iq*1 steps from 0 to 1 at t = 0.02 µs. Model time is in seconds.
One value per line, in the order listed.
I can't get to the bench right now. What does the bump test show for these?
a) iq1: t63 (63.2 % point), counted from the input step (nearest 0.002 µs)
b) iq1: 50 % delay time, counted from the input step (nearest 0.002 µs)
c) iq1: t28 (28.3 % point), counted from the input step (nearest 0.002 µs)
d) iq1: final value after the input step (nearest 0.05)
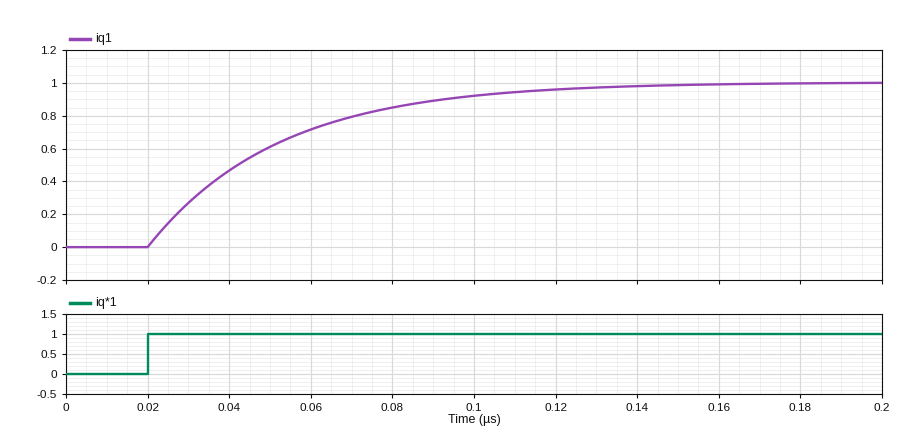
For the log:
0.032 µs
0.022 µs
0.010 µs
1.00
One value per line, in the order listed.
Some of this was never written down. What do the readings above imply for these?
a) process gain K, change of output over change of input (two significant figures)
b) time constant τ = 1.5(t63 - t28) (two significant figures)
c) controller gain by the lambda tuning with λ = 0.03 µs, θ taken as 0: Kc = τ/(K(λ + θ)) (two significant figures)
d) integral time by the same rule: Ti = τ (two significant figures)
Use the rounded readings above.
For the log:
1.0
0.033 µs
1.1
0.033 µs
